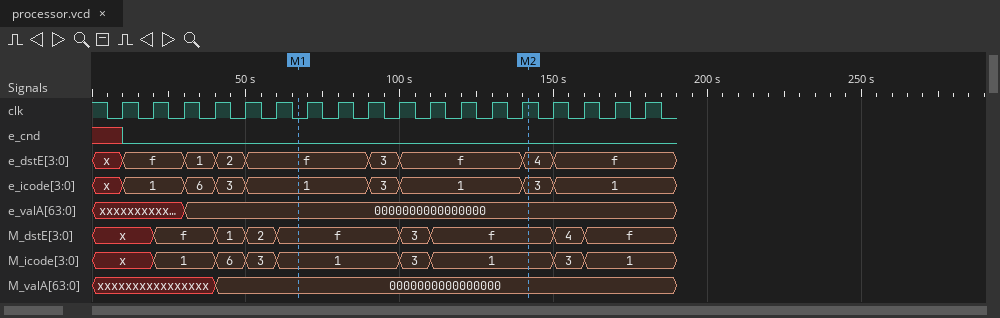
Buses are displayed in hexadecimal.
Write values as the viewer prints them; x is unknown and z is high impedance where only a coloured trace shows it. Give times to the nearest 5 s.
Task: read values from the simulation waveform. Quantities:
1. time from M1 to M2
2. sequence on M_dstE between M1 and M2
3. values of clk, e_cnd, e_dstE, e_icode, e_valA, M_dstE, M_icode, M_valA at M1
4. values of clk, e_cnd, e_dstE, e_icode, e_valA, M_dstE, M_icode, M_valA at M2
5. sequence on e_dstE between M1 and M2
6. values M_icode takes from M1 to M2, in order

75 s
f, 3, f
clk=0, e_cnd=0, e_dstE=f, e_icode=1, e_valA=0000000000000000, M_dstE=f, M_icode=1, M_valA=0000000000000000
clk=1, e_cnd=0, e_dstE=4, e_icode=3, e_valA=0000000000000000, M_dstE=f, M_icode=1, M_valA=0000000000000000
f, 3, f, 4
1, 3, 1
